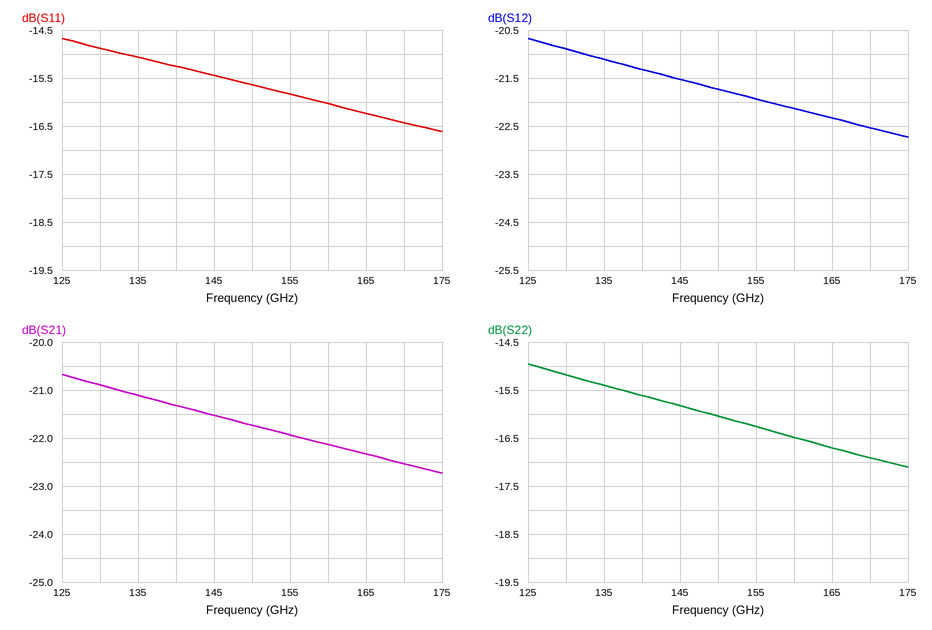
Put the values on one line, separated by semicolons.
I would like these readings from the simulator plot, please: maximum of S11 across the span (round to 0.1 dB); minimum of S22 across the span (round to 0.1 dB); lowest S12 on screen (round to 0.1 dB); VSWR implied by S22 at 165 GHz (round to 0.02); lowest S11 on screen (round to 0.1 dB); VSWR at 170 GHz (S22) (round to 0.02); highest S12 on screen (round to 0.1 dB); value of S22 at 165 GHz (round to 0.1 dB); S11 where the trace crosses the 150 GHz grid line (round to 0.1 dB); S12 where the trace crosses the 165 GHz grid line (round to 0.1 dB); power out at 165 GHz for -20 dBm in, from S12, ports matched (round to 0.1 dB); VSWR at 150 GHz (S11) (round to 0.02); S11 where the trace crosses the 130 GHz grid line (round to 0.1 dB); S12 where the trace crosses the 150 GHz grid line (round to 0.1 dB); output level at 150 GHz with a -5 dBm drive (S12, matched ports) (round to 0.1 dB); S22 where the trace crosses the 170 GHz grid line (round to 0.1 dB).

-14.7 dB; -17.1 dB; -22.7 dB; 1.34; -16.6 dB; 1.34; -20.7 dB; -16.7 dB; -15.6 dB; -22.3 dB; -42.3 dBm; 1.40; -14.9 dB; -21.7 dB; -26.7 dBm; -16.9 dB
